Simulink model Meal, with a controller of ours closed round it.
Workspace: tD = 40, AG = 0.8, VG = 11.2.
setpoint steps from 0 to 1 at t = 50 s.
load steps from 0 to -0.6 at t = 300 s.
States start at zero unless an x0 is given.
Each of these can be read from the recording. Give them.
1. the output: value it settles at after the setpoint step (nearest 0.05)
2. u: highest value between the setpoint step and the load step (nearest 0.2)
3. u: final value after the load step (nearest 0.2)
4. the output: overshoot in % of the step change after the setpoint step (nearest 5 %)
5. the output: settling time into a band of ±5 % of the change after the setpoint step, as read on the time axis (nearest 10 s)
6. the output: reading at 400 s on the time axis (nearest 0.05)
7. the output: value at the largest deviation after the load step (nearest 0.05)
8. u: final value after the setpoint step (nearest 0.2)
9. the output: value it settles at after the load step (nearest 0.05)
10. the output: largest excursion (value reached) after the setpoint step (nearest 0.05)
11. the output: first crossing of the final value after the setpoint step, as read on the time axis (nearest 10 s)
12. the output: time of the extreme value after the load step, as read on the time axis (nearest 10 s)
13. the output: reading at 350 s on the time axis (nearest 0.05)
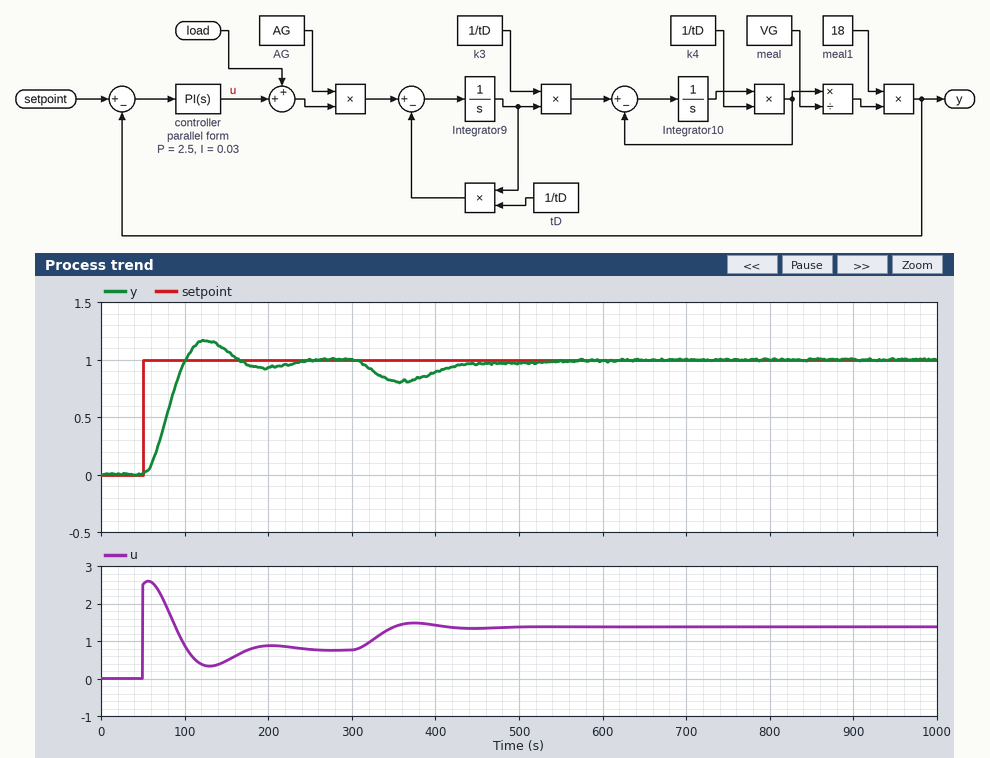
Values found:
1.00
2.6
1.4
15 %
220 s
0.90
0.80
0.8
1.00
1.15
100 s
360 s
0.80
